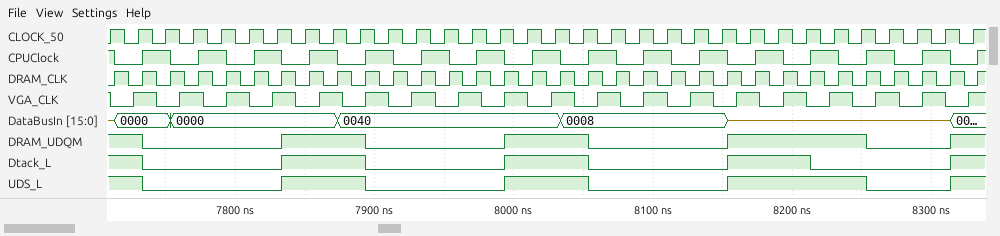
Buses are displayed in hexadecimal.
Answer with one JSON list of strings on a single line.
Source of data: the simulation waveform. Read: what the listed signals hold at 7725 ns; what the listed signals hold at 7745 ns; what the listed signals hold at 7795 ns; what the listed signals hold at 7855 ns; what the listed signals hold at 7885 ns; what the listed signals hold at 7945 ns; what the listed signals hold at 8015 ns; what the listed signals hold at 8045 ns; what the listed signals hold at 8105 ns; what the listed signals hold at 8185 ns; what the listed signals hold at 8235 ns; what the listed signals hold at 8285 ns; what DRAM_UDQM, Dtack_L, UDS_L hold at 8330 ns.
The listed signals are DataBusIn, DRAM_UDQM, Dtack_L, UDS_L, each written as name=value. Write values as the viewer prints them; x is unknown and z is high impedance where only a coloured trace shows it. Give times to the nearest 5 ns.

["DataBusIn=0000, DRAM_UDQM=1, Dtack_L=1, UDS_L=1", "DataBusIn=0000, DRAM_UDQM=0, Dtack_L=0, UDS_L=0", "DataBusIn=0000, DRAM_UDQM=0, Dtack_L=0, UDS_L=0", "DataBusIn=0000, DRAM_UDQM=1, Dtack_L=1, UDS_L=1", "DataBusIn=0040, DRAM_UDQM=1, Dtack_L=1, UDS_L=1", "DataBusIn=0040, DRAM_UDQM=0, Dtack_L=0, UDS_L=0", "DataBusIn=0040, DRAM_UDQM=1, Dtack_L=1, UDS_L=1", "DataBusIn=0008, DRAM_UDQM=1, Dtack_L=1, UDS_L=1", "DataBusIn=0008, DRAM_UDQM=0, Dtack_L=0, UDS_L=0", "DataBusIn=z, DRAM_UDQM=1, Dtack_L=1, UDS_L=1", "DataBusIn=z, DRAM_UDQM=1, Dtack_L=0, UDS_L=1", "DataBusIn=z, DRAM_UDQM=0, Dtack_L=0, UDS_L=0", "DRAM_UDQM=1, Dtack_L=1, UDS_L=1"]
